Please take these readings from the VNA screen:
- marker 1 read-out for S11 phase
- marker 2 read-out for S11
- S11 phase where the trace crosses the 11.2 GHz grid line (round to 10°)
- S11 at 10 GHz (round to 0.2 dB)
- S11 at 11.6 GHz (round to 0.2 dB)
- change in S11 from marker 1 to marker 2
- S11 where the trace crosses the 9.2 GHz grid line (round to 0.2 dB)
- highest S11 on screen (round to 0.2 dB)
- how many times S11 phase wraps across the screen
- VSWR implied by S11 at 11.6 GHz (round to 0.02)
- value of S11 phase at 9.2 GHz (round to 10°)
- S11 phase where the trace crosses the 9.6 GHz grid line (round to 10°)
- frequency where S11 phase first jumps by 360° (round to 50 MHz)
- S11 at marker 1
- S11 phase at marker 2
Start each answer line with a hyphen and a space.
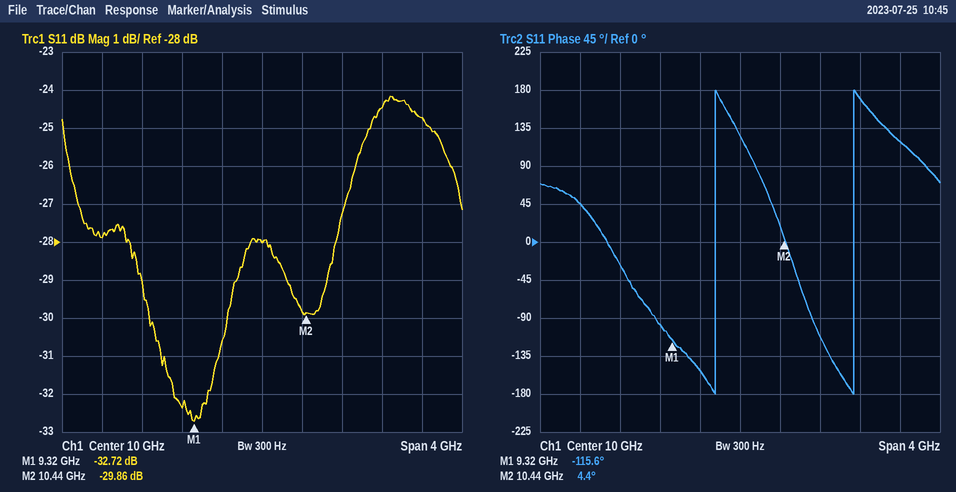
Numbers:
- -115.6°
- -29.86 dB
- 170°
- -28.0 dB
- -24.8 dB
- 2.86 dB
- -32.4 dB
- -24.2 dB
- 2
- 1.12
- -100°
- -150°
- 9.75 GHz
- -32.72 dB
- 4.4°
